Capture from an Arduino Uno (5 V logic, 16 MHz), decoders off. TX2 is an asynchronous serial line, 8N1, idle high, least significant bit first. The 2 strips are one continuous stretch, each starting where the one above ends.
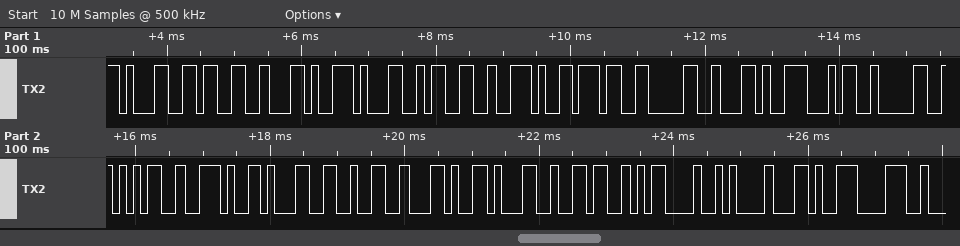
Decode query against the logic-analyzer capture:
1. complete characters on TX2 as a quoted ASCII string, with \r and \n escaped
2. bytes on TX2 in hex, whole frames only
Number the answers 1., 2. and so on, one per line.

1. "13,13.70,405.12,16\r\n,8"
2. 31 33 2C 31 33 2E 37 30 2C 34 30 35 2E 31 32 2C 31 36 0D 0A 2C 38
